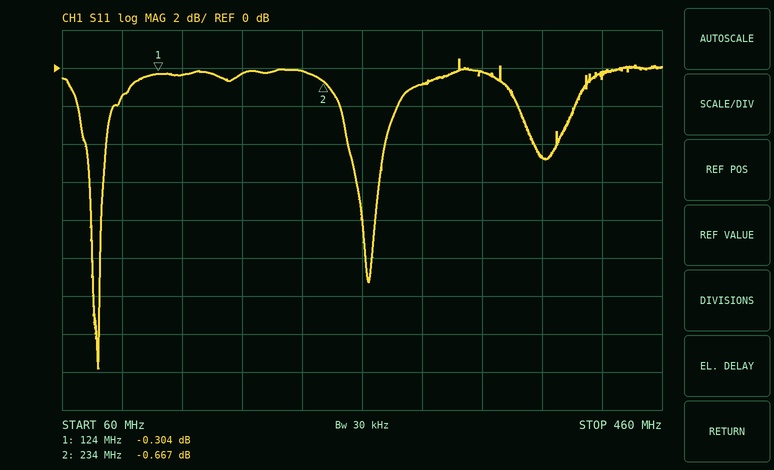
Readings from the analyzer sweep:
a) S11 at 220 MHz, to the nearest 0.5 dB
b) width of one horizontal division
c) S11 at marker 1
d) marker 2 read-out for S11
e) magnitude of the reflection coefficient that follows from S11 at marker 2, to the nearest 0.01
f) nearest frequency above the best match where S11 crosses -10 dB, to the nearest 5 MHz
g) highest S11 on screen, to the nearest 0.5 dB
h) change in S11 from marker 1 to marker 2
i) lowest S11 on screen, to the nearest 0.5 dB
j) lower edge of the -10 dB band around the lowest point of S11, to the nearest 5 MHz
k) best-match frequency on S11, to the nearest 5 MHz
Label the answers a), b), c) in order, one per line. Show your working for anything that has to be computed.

a) 0.0 dB
b) 40 MHz
c) -0.304 dB
d) -0.667 dB
e) 10^(-0.667/20) ≈ 0.93
f) 85 MHz
g) 0.5 dB
h) -0.667 − (-0.304) = -0.363 dB
i) -16.0 dB
j) 80 MHz
k) 85 MHz
